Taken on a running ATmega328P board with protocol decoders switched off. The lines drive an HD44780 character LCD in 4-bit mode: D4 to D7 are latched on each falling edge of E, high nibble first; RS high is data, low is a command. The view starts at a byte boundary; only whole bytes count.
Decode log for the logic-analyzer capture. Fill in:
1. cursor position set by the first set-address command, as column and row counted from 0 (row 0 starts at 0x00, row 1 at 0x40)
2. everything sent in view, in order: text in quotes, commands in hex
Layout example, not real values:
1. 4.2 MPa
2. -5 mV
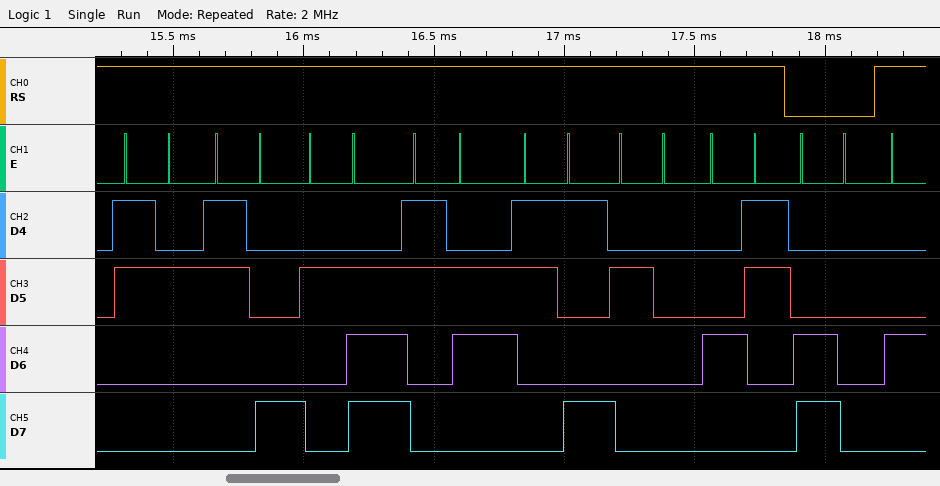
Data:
1. column 0, row 1
2. "28.69 C" 0xC0
